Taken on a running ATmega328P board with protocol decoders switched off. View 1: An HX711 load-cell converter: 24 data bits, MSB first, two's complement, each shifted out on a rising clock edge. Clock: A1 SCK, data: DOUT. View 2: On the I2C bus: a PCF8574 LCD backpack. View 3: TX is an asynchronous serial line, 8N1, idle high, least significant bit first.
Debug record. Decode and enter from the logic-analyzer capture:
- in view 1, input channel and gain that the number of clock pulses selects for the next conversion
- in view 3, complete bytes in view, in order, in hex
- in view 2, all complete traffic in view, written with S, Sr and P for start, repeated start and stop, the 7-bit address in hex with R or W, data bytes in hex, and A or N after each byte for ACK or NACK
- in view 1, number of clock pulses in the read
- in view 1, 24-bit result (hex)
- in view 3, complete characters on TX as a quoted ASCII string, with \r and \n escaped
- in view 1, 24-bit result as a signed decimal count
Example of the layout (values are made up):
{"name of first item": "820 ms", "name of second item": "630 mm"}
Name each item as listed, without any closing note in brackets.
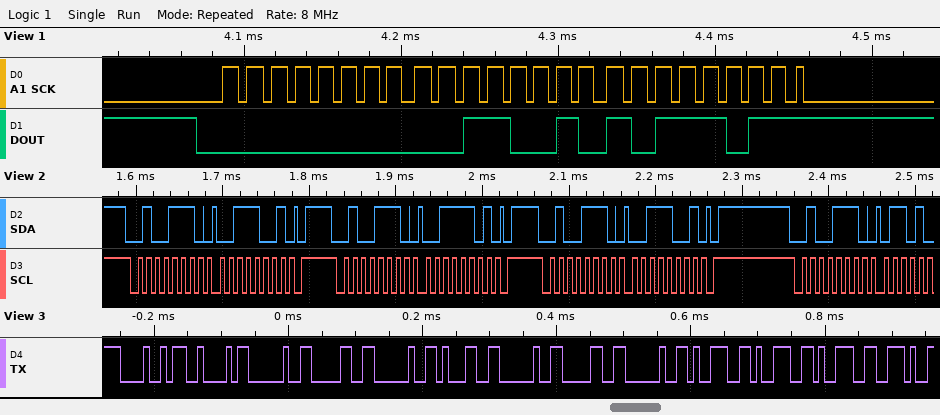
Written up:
{"in view 1, input channel and gain that the number of clock pulses selects for the next conversion": "channel A, gain 128", "in view 3, complete bytes in view, in order, in hex": "48 42 20 30 20 31 20 30 20 39 39 39 2E", "in view 2, all complete traffic in view, written with S, Sr and P for start, repeated start and stop, the 7-bit address in hex with R or W, data bytes in hex, and A or N after each byte for ACK or NACK": "S 27W A 39 A P S 27W A 3D A P S 27W A 39 A P S 27W A", "in view 1, number of clock pulses in the read": "25", "in view 1, 24-bit result": "0x0032BB", "in view 3, complete characters on TX as a quoted ASCII string, with \\r and \\n escaped": "\"HB 0 1 0 999.\"", "in view 1, 24-bit result as a signed decimal count": "12987"}
